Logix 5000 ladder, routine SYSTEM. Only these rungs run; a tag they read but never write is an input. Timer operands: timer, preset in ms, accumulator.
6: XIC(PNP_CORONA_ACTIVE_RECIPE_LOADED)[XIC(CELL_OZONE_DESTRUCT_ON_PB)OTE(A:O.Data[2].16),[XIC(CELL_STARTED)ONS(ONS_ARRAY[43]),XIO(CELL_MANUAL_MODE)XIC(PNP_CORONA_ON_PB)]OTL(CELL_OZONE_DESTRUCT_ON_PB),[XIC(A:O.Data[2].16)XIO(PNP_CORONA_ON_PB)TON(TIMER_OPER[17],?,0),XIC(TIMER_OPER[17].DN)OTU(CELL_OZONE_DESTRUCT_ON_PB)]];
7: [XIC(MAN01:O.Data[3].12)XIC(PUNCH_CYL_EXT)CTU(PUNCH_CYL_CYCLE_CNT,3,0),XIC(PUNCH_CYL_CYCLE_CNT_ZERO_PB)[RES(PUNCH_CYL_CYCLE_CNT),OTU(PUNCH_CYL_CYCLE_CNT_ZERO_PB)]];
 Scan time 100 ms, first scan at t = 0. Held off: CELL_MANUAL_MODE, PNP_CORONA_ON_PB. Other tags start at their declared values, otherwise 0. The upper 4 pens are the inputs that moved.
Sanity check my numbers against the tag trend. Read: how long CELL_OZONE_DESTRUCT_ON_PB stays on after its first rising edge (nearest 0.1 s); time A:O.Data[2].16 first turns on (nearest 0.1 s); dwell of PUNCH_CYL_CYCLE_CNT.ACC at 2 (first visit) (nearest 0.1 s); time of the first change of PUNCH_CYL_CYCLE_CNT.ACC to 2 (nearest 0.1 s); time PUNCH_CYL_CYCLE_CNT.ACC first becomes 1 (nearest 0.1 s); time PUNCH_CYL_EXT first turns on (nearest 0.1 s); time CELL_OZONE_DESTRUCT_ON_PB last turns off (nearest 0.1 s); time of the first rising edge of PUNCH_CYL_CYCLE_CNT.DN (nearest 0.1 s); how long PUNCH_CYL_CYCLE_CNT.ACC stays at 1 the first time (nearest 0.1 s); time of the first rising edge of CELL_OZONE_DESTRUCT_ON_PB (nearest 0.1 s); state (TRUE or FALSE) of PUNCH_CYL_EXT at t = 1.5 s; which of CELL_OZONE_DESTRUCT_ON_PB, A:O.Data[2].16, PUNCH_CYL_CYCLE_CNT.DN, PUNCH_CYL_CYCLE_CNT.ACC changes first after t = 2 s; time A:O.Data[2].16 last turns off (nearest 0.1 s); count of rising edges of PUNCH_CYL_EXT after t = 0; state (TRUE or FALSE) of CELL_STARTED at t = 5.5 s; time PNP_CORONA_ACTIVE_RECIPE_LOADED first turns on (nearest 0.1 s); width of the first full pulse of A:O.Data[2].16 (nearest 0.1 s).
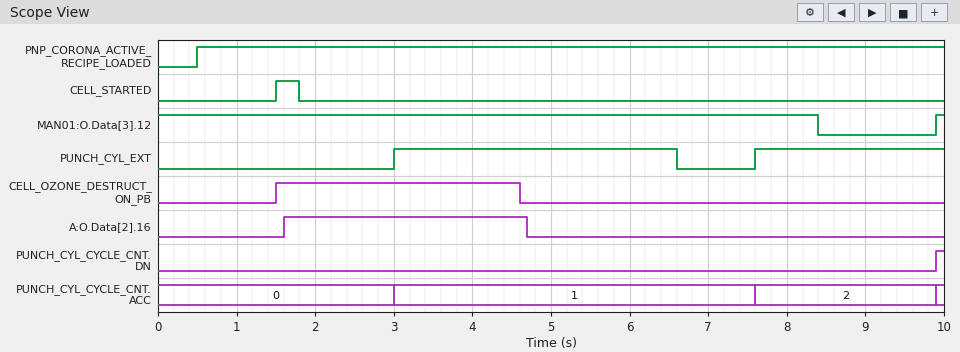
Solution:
3.1 s
1.6 s
2.3 s
7.6 s
3.0 s
3.0 s
4.6 s
9.9 s
4.6 s
1.5 s
FALSE
PUNCH_CYL_CYCLE_CNT.ACC
4.7 s
2
FALSE
0.5 s
3.1 s
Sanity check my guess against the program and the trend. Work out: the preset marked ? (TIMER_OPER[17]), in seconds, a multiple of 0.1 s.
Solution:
3.0 s
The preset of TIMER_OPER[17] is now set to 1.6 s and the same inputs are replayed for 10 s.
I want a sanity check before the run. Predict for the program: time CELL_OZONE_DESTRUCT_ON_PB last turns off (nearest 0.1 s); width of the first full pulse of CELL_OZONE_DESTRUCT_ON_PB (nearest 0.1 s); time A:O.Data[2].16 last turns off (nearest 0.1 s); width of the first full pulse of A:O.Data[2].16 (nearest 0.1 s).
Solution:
3.2 s
1.7 s
3.3 s
1.7 s
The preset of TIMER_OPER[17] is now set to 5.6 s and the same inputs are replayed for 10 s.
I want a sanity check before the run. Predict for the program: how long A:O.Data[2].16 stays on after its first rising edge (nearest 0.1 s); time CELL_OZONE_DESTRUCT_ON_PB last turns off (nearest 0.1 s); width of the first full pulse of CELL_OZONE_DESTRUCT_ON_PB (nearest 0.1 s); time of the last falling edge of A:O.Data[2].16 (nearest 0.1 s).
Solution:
5.7 s
7.2 s
5.7 s
7.3 s
